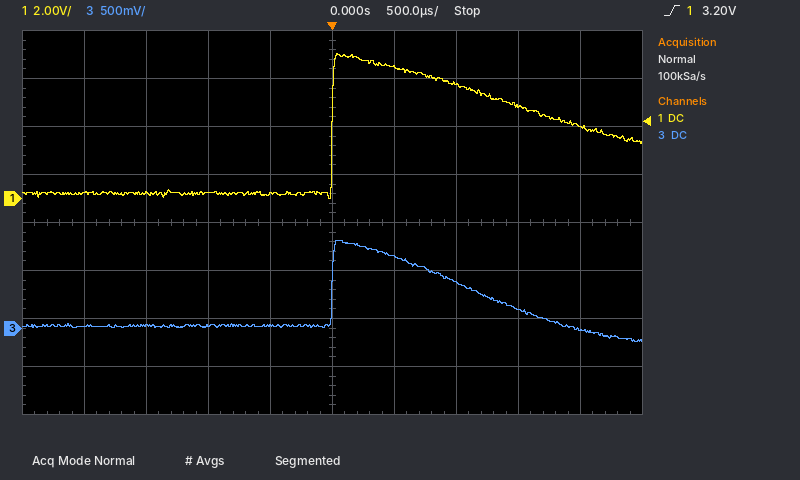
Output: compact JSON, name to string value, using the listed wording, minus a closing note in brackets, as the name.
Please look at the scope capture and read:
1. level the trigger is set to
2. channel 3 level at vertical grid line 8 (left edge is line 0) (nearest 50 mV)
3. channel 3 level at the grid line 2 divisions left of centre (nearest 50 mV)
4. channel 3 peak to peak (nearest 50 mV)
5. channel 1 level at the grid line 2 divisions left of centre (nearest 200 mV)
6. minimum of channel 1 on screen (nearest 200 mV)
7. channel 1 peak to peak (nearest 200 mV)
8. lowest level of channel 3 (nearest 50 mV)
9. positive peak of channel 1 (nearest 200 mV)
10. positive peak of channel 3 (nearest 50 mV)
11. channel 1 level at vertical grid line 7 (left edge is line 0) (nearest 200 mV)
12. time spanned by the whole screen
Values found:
{"level the trigger is set to": "3.20 V", "channel 3 level at vertical grid line 8 (left edge is line 0)": "200 mV", "channel 3 level at the grid line 2 divisions left of centre": "0 mV", "channel 3 peak to peak": "1.05 V", "channel 1 level at the grid line 2 divisions left of centre": "200 mV", "minimum of channel 1 on screen": "0.0 V", "channel 1 peak to peak": "6.0 V", "lowest level of channel 3": "-150 mV", "positive peak of channel 1": "6.0 V", "positive peak of channel 3": "900 mV", "channel 1 level at vertical grid line 7 (left edge is line 0)": "4.8 V", "time spanned by the whole screen": "5 ms"}
